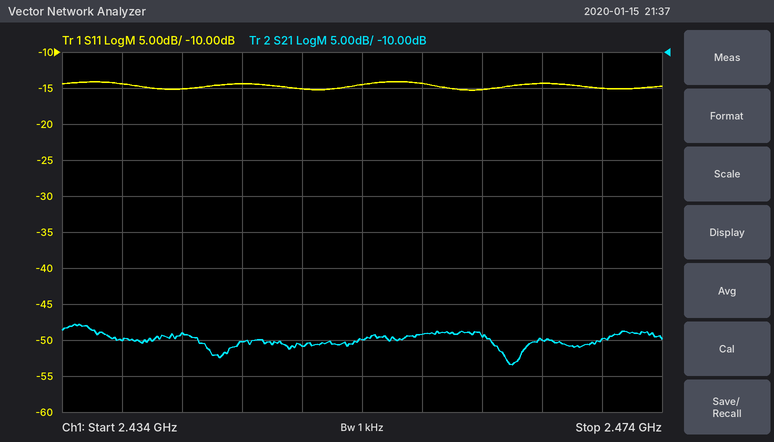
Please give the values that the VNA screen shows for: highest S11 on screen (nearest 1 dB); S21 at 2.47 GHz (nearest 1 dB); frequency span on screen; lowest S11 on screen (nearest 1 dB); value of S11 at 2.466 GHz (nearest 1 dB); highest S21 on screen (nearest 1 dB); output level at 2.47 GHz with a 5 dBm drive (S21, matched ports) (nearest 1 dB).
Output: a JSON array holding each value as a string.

["-14 dB", "-50 dB", "40 MHz", "-15 dB", "-14 dB", "-48 dB", "-45 dBm"]
